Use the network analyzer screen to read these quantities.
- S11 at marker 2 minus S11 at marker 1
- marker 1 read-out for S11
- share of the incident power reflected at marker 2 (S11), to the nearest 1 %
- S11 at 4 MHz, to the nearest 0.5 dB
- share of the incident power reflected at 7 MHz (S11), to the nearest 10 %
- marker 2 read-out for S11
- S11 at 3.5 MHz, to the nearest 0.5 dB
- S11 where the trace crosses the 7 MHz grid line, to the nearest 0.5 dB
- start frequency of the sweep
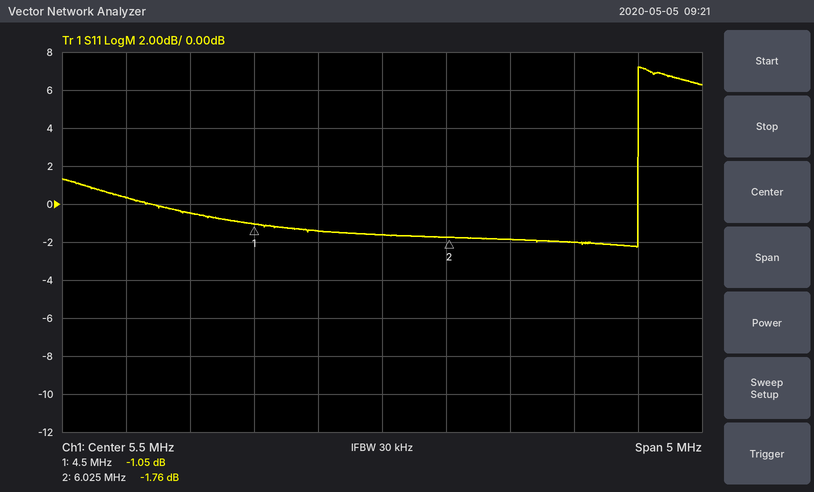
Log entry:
-0.71 dB
-1.05 dB
67 %
-0.5 dB
60 %
-1.76 dB
0.5 dB
-2.0 dB
3 MHz
